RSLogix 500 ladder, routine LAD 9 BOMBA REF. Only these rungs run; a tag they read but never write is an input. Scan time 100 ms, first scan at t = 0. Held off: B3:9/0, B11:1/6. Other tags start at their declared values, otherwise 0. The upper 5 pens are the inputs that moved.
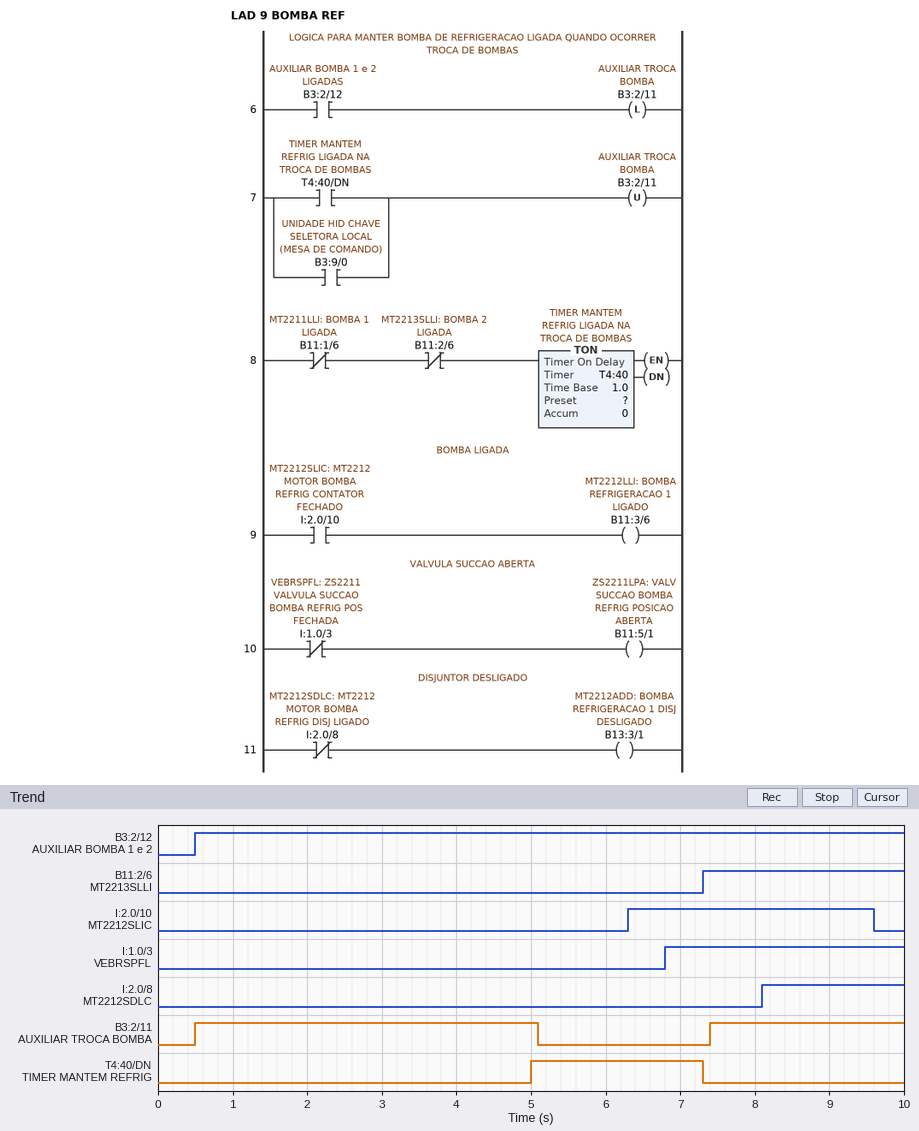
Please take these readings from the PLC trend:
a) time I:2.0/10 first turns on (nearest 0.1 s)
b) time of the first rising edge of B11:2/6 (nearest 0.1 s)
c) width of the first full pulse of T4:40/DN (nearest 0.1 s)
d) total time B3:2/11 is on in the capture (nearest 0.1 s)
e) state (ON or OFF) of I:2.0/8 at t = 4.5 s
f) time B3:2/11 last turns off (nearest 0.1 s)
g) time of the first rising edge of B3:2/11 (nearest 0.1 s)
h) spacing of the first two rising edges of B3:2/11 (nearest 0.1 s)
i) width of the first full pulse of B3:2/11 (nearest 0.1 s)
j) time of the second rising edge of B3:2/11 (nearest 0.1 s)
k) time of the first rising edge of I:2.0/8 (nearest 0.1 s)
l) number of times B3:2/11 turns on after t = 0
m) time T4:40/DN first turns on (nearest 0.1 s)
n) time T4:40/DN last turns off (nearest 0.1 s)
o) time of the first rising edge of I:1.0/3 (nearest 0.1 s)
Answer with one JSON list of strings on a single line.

["6.3 s", "7.3 s", "2.3 s", "7.2 s", "OFF", "5.1 s", "0.5 s", "6.9 s", "4.6 s", "7.4 s", "8.1 s", "2", "5.0 s", "7.3 s", "6.8 s"]
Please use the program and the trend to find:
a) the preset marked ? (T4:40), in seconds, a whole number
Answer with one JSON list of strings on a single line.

["5 s"]
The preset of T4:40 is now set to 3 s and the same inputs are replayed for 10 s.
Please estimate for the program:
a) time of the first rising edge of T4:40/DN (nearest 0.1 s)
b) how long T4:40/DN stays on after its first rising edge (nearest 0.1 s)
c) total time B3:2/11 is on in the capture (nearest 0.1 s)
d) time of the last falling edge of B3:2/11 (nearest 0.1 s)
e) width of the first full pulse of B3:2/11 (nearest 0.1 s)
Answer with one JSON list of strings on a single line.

["3.0 s", "4.3 s", "5.2 s", "3.1 s", "2.6 s"]
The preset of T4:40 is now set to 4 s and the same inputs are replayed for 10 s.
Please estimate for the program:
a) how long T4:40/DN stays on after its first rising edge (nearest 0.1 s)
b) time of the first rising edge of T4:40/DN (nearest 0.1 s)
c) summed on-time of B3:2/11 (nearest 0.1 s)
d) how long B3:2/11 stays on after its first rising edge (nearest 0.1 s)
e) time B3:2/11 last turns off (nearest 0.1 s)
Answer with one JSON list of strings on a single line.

["3.3 s", "4.0 s", "6.2 s", "3.6 s", "4.1 s"]
